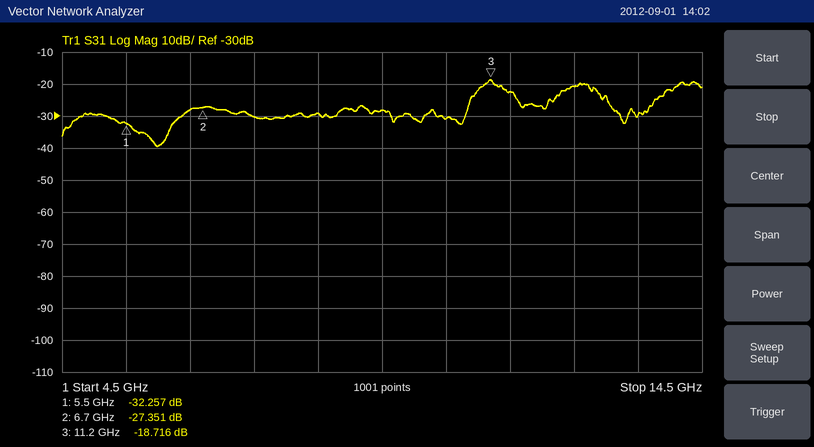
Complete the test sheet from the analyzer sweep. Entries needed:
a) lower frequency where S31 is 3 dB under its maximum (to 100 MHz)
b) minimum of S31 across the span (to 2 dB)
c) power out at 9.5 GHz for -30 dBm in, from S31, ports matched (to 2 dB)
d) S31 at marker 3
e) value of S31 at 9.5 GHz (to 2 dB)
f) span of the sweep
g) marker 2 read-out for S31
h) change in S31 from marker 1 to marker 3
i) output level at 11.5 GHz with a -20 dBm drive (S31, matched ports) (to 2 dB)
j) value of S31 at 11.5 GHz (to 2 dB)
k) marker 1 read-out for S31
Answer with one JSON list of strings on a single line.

["11.0 GHz", "-40 dB", "-58 dBm", "-18.716 dB", "-28 dB", "10 GHz", "-27.351 dB", "13.541 dB", "-42 dBm", "-22 dB", "-32.257 dB"]
